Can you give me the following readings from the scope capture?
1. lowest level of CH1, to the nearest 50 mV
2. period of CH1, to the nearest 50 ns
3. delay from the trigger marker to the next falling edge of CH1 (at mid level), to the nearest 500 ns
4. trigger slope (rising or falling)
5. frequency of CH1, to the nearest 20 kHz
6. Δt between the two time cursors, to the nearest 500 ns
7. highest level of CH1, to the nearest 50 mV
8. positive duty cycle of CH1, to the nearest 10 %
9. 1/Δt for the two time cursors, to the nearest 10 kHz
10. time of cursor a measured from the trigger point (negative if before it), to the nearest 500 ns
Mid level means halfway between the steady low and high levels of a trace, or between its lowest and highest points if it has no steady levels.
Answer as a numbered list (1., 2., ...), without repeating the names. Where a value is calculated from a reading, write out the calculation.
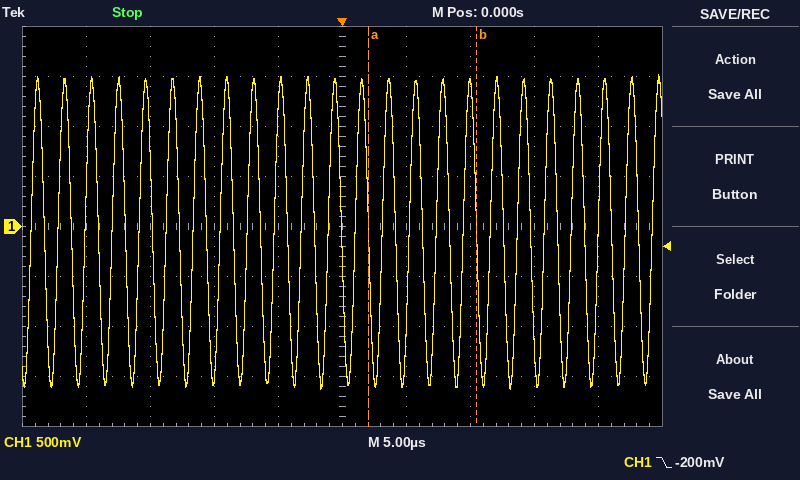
1. -1.60 V
2. 2.10 µs
3. 2.0 µs
4. falling
5. 1 / 2.10 µs ≈ 476 kHz, so 480 kHz to the nearest 20 kHz
6. 8.5 µs
7. 1.50 V
8. 50 %
9. 1 / 8.5 µs ≈ 120 kHz
10. +2.0 µs
